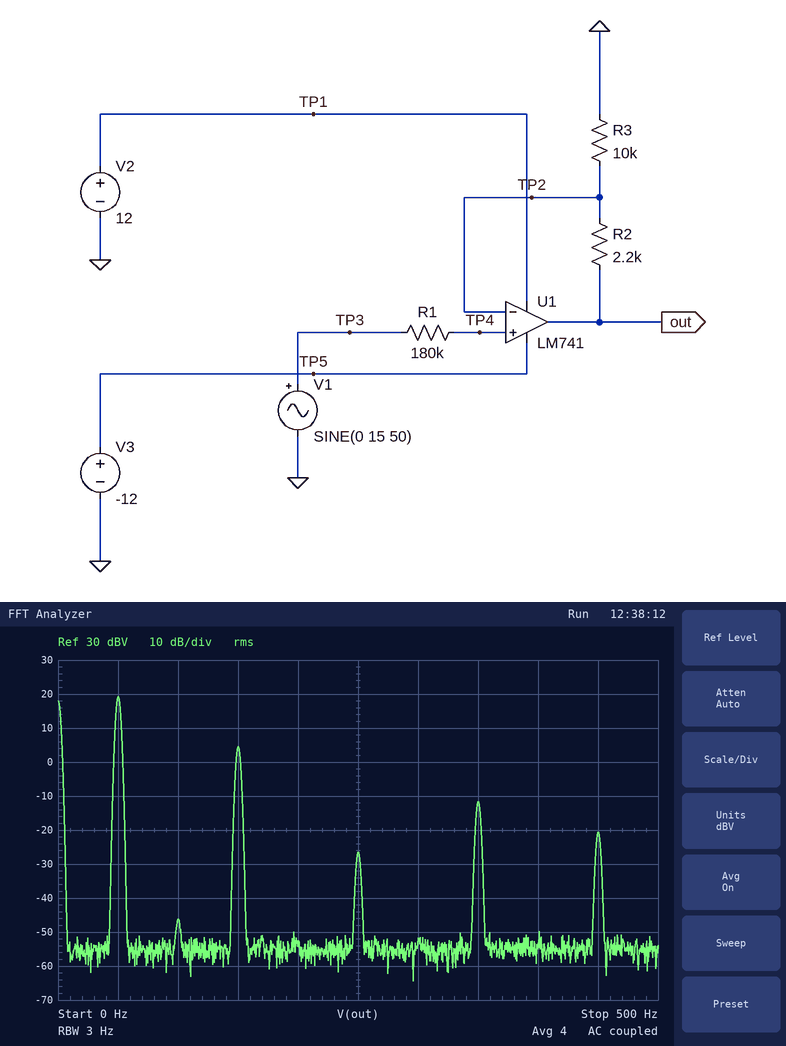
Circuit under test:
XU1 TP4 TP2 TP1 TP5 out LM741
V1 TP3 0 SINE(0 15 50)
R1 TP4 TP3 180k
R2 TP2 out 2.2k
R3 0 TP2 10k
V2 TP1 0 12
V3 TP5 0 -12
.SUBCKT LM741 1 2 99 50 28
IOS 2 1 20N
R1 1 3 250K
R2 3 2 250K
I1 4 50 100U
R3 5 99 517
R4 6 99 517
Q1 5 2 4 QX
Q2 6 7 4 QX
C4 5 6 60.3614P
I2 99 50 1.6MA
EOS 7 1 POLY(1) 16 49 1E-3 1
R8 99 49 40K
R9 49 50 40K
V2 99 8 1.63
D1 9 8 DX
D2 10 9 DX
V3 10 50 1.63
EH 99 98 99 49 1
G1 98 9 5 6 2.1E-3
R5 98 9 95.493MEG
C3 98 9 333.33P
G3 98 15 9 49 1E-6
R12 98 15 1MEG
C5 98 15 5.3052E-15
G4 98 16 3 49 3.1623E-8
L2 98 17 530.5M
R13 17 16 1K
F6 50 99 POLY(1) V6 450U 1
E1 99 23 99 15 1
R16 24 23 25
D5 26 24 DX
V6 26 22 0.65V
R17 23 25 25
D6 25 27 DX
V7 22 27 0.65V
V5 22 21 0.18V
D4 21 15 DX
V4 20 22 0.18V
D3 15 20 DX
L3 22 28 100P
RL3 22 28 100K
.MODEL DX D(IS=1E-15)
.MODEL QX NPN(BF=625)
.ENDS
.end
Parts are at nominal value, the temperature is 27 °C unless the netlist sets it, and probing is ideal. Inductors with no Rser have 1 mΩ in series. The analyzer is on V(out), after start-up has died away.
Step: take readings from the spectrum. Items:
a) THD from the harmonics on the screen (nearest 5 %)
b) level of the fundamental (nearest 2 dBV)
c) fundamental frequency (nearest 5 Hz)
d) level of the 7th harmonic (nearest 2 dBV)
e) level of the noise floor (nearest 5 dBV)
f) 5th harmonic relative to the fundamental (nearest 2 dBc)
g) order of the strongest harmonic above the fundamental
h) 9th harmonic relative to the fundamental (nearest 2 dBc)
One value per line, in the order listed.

20 %
20 dBV
50 Hz
-12 dBV
-55 dBV
-46 dBc
3
-40 dBc
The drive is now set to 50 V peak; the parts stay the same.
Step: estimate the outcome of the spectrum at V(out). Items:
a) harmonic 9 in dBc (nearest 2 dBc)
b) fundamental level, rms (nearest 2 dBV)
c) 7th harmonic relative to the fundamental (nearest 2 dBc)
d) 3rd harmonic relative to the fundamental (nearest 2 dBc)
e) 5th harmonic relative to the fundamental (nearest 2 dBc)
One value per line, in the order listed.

-20 dBc
10 dBV
-18 dBc
6 dBc
0 dBc
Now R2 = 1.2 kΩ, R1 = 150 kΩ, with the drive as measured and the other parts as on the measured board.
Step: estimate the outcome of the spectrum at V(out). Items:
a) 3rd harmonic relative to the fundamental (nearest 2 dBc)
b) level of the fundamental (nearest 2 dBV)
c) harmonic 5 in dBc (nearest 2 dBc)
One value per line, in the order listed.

-16 dBc
20 dBV
-38 dBc
